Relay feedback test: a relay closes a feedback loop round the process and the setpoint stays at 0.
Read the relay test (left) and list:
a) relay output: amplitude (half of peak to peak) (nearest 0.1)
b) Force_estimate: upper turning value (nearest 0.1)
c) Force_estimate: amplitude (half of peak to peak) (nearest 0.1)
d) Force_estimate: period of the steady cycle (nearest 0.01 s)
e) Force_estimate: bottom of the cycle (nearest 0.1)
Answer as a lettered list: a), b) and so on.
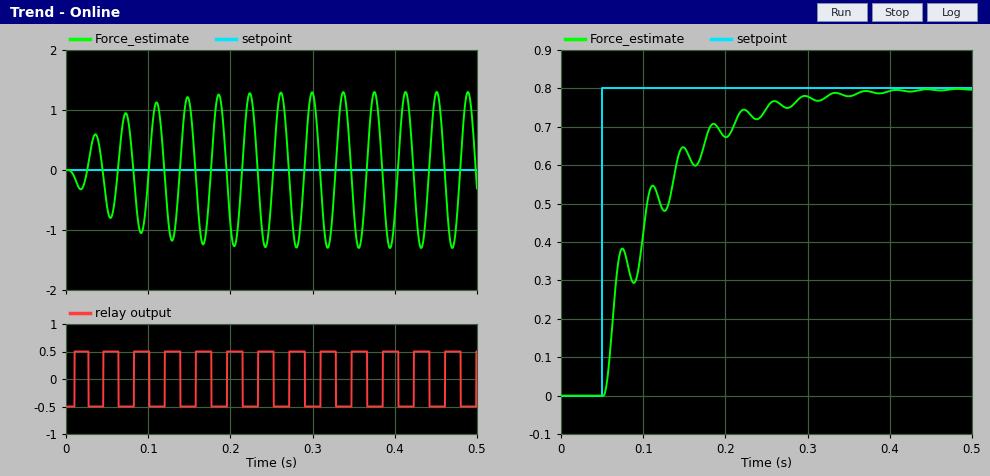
a) 0.5
b) 1.3
c) 1.3
d) 0.04 s
e) -1.3
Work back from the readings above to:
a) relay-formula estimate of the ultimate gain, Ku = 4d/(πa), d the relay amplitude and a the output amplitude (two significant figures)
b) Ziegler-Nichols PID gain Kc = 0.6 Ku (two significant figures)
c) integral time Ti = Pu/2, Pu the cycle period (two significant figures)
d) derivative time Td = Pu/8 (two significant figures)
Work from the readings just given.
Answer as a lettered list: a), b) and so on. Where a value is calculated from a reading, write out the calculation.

a) 4 × 0.5 / (π × 1.3) = 0.49
b) 0.6 × 0.49 = 0.29
c) 0.04 / 2 = 0.020 s
d) 0.04 / 8 = 0.0050 s
